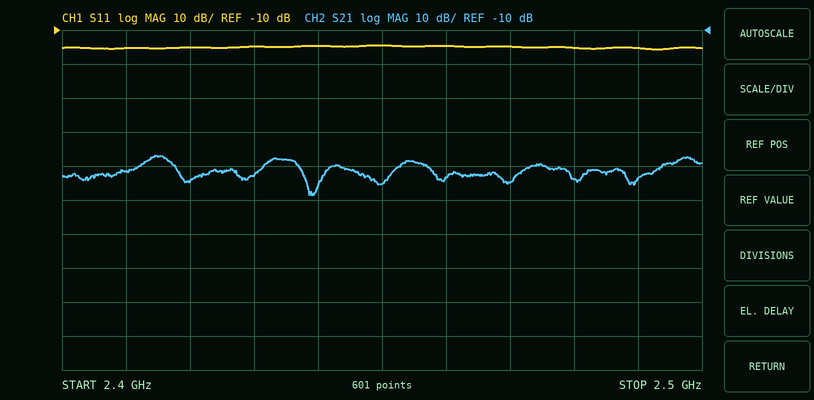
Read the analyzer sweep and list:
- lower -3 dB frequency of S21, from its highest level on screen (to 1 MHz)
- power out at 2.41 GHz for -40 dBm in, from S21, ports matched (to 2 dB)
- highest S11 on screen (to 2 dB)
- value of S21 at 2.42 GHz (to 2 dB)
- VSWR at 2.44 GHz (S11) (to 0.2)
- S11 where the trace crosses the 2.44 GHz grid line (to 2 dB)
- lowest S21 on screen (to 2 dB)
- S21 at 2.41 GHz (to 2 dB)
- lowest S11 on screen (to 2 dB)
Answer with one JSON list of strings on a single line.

["2.412 GHz", "-92 dBm", "-14 dB", "-54 dB", "1.4", "-14 dB", "-58 dB", "-52 dB", "-16 dB"]
